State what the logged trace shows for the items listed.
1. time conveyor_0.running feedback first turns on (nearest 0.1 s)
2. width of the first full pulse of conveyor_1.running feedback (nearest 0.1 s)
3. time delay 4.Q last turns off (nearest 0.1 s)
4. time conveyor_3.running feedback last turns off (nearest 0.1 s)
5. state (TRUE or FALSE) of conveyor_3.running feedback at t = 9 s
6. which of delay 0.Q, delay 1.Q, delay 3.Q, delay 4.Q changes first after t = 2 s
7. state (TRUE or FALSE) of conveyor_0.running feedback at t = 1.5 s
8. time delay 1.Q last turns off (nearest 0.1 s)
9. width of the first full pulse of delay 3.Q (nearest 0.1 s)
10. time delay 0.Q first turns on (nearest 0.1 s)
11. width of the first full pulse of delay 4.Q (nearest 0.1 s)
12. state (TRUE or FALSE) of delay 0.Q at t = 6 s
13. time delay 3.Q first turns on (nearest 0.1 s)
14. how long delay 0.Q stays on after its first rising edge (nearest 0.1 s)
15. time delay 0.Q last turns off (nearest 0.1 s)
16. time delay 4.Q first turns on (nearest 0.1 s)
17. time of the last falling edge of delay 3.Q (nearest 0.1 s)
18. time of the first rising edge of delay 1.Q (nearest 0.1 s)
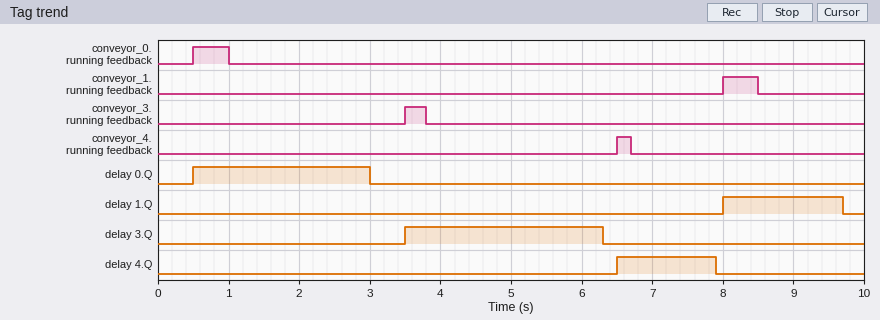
0.5 s
0.5 s
7.9 s
3.8 s
FALSE
delay 0.Q
FALSE
9.7 s
2.8 s
0.5 s
1.4 s
FALSE
3.5 s
2.5 s
3.0 s
6.5 s
6.3 s
8.0 s
